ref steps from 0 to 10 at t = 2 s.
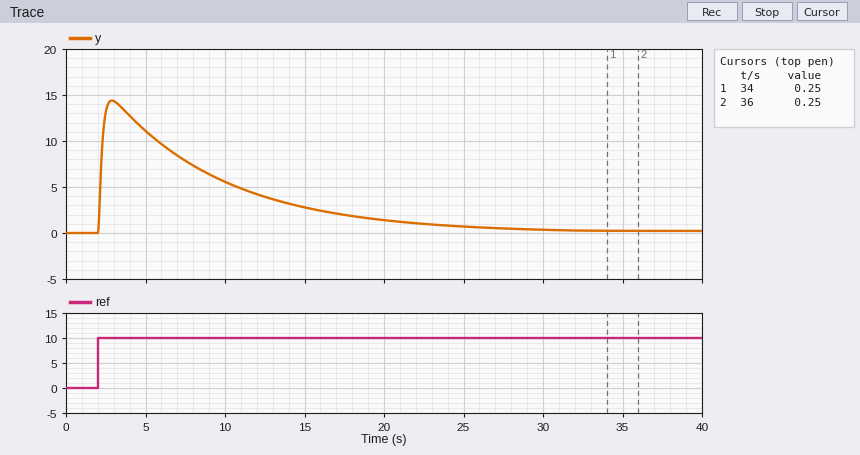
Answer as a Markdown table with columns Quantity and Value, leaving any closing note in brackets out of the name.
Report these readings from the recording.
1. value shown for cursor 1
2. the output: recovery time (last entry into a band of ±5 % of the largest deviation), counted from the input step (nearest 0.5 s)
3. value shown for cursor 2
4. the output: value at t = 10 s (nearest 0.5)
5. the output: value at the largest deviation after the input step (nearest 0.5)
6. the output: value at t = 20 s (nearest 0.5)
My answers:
| Quantity | Value |
|---|---|
| value shown for cursor 1 | 0.25 |
| the output: recovery time (last entry into a band of ±5 % of the largest deviation), counted from the input step | 21.0 s |
| value shown for cursor 2 | 0.25 |
| the output: value at t = 10 s | 5.5 |
| the output: value at the largest deviation after the input step | 14.5 |
| the output: value at t = 20 s | 1.5 |
